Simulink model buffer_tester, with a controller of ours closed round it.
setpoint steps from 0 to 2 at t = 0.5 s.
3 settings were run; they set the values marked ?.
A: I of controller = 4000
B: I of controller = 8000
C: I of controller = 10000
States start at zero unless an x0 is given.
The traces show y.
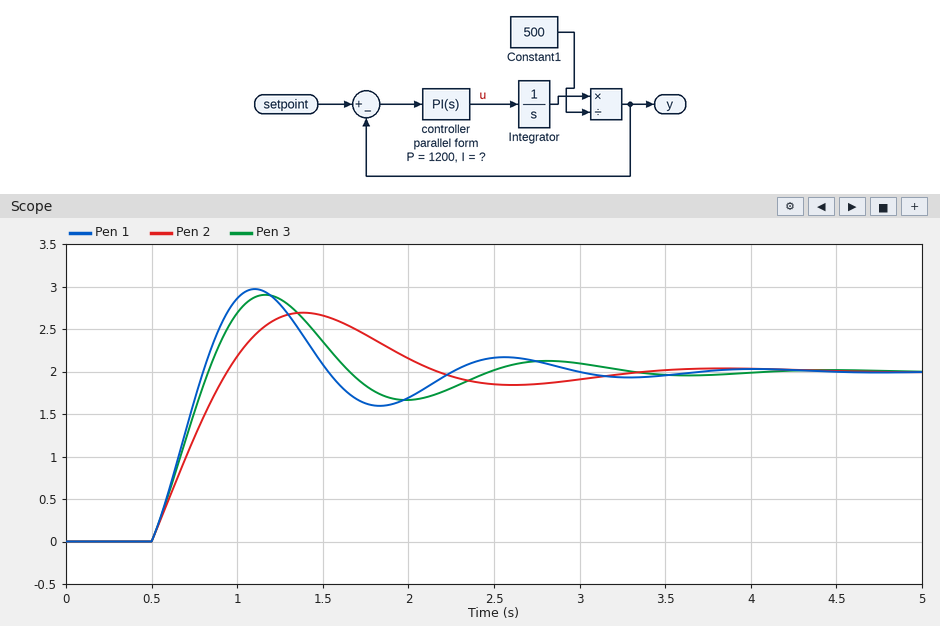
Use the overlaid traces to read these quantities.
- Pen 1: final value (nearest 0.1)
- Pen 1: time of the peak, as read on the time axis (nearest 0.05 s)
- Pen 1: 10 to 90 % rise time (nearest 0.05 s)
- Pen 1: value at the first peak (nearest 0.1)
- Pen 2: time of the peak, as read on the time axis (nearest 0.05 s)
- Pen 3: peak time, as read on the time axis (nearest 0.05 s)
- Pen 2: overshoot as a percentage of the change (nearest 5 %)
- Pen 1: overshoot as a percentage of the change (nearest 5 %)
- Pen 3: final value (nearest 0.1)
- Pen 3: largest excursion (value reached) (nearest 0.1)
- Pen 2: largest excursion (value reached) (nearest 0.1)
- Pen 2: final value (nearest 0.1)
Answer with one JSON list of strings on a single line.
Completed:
["2.0", "1.10 s", "0.25 s", "3.0", "1.40 s", "1.15 s", "35 %", "50 %", "2.0", "2.9", "2.7", "2.0"]
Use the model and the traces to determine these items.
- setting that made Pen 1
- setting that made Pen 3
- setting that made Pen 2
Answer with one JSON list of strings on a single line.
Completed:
["C", "B", "A"]
